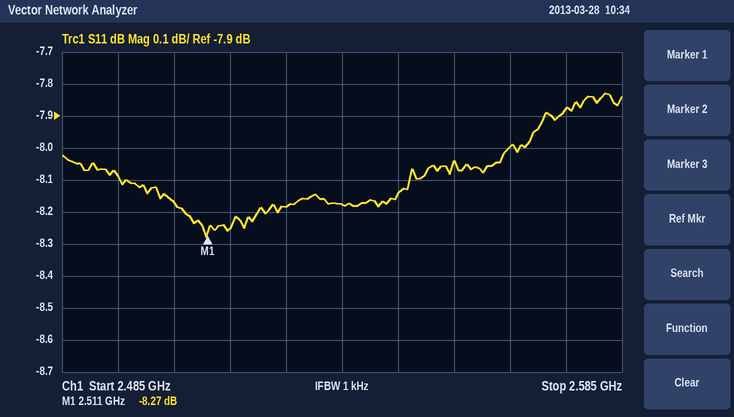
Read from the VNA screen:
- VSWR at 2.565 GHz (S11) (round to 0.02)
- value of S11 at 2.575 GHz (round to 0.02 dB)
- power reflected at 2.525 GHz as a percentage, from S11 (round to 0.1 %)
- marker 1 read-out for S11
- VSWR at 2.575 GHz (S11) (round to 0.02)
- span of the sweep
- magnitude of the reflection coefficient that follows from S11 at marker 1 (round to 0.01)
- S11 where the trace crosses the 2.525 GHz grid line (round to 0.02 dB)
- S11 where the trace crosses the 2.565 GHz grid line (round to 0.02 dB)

2.32
-7.88 dB
15.2 %
-8.27 dB
2.36
100 MHz
0.39
-8.18 dB
-8.00 dB
